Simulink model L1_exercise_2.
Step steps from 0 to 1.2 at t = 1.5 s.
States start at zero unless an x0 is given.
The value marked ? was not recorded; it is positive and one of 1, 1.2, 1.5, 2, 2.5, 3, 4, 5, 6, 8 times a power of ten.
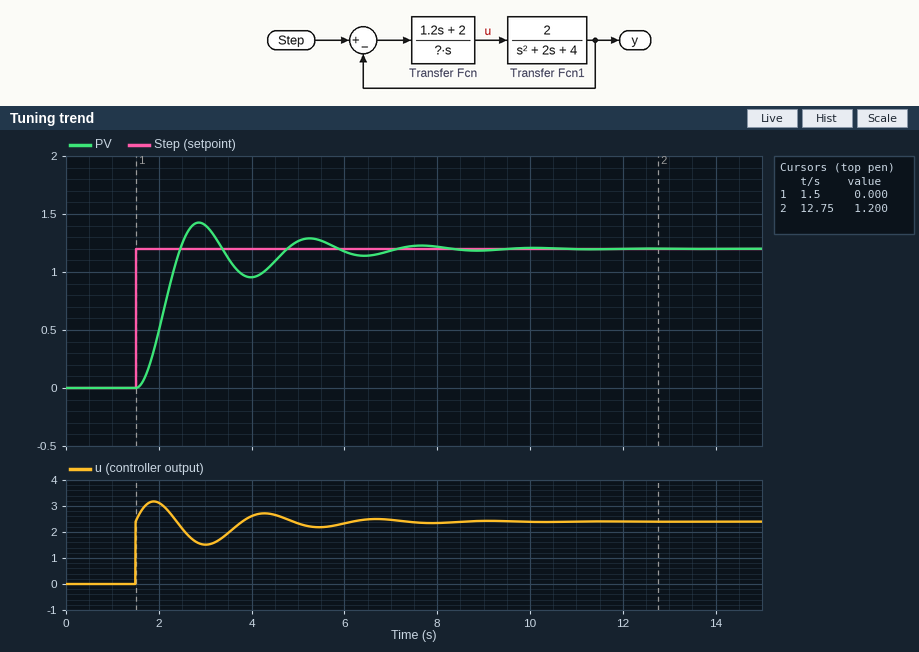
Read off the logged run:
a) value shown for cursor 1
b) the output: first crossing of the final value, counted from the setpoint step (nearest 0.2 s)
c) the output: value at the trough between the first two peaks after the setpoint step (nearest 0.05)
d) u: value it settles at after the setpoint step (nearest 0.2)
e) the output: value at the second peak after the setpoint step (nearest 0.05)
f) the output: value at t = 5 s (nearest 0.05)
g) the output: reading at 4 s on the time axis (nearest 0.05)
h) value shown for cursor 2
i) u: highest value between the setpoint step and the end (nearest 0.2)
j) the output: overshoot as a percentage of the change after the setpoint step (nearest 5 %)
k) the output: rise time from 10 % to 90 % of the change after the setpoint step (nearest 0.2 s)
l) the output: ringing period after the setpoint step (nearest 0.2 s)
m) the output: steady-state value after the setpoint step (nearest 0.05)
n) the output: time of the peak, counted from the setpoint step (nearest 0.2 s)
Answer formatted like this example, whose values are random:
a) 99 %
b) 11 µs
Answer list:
a) 0.000
b) 1.0 s
c) 0.95
d) 2.4
e) 1.30
f) 1.25
g) 0.95
h) 1.200
i) 3.2
j) 20 %
k) 0.6 s
l) 2.4 s
m) 1.20
n) 1.4 s
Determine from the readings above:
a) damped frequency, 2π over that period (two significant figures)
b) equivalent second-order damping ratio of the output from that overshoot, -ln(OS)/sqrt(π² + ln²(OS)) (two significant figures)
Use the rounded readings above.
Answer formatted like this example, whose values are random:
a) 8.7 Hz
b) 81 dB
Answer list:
a) 2.6 rad/s
b) 0.46
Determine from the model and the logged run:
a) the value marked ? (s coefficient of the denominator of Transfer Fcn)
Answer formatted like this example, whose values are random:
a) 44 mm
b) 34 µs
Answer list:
a) 0.6
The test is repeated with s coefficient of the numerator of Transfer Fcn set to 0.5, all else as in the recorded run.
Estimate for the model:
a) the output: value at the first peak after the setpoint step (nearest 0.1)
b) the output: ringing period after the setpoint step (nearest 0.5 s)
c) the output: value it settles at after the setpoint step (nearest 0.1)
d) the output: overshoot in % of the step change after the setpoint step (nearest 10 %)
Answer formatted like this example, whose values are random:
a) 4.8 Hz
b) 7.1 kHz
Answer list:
a) 1.6
b) 3.0 s
c) 1.2
d) 30 %
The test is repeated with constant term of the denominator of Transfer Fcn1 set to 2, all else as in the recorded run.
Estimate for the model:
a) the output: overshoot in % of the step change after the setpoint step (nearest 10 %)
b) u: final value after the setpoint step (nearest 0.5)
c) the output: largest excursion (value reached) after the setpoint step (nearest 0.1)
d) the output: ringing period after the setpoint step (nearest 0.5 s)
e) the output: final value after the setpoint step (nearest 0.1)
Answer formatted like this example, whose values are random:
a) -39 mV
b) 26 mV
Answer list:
a) 50 %
b) 1.0
c) 1.8
d) 3.0 s
e) 1.2
